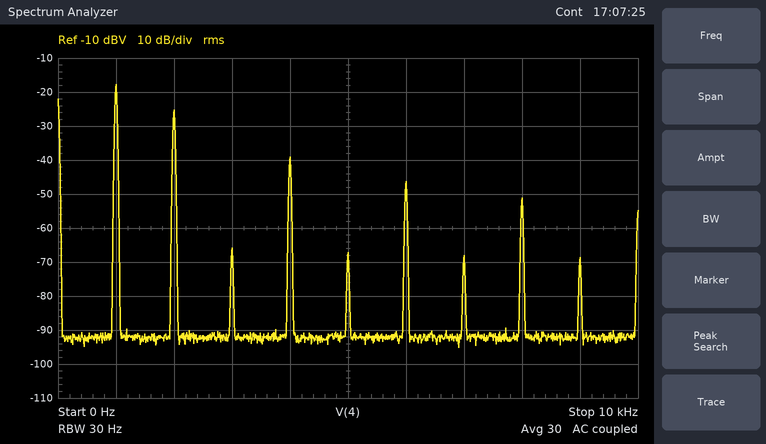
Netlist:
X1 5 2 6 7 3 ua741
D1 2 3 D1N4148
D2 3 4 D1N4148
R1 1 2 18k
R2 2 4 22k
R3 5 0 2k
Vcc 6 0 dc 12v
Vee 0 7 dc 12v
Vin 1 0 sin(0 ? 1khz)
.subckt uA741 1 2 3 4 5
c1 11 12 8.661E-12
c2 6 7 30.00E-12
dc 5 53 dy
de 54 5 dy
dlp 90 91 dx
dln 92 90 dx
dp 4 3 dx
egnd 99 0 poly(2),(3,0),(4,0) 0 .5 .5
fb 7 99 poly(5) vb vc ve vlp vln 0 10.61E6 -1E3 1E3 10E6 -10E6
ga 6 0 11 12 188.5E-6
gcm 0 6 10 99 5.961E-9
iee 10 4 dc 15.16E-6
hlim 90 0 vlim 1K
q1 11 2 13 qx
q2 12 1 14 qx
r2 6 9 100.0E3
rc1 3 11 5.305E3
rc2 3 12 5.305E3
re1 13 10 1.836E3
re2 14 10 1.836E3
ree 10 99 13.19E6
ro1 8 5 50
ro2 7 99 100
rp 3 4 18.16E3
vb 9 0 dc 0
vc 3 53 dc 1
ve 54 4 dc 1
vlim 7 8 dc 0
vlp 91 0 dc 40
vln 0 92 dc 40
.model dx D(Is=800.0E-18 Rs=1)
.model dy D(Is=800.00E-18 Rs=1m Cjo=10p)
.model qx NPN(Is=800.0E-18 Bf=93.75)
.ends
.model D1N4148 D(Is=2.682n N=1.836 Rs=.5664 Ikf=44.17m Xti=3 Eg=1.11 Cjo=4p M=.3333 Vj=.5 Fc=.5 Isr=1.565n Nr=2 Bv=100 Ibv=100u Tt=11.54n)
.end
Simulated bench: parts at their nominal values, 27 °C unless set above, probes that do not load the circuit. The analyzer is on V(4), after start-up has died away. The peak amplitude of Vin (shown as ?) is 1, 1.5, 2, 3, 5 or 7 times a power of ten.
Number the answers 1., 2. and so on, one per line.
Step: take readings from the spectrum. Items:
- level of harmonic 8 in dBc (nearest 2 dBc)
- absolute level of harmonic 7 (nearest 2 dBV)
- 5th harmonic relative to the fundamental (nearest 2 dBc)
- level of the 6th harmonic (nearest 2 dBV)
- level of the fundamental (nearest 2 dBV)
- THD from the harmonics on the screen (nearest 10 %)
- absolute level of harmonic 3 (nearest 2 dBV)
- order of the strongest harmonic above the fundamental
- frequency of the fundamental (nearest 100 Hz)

1. -34 dBc
2. -68 dBV
3. -50 dBc
4. -46 dBV
5. -18 dBV
6. 40 %
7. -66 dBV
8. 2
9. 1.0 kHz
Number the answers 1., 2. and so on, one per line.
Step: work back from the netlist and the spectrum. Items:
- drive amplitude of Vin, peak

1. 300 mV
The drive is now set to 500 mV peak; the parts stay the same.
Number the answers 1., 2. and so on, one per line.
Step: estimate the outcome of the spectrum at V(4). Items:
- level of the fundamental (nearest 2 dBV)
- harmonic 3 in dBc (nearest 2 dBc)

1. -14 dBV
2. -52 dBc
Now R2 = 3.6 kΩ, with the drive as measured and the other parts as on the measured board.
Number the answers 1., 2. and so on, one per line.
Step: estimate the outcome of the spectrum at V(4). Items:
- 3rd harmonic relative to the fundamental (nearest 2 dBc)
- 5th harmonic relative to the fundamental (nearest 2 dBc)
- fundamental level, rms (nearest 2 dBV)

1. -36 dBc
2. -38 dBc
3. -34 dBV
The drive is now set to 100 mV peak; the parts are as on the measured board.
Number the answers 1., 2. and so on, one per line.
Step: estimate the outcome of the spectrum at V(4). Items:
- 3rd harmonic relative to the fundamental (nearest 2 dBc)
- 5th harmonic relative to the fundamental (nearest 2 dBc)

1. -40 dBc
2. -42 dBc
